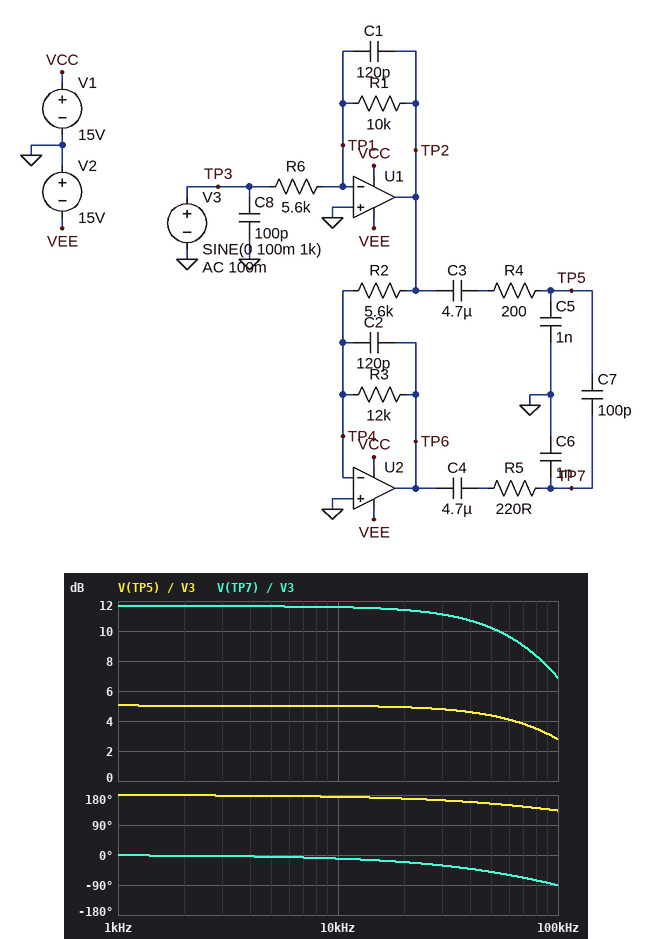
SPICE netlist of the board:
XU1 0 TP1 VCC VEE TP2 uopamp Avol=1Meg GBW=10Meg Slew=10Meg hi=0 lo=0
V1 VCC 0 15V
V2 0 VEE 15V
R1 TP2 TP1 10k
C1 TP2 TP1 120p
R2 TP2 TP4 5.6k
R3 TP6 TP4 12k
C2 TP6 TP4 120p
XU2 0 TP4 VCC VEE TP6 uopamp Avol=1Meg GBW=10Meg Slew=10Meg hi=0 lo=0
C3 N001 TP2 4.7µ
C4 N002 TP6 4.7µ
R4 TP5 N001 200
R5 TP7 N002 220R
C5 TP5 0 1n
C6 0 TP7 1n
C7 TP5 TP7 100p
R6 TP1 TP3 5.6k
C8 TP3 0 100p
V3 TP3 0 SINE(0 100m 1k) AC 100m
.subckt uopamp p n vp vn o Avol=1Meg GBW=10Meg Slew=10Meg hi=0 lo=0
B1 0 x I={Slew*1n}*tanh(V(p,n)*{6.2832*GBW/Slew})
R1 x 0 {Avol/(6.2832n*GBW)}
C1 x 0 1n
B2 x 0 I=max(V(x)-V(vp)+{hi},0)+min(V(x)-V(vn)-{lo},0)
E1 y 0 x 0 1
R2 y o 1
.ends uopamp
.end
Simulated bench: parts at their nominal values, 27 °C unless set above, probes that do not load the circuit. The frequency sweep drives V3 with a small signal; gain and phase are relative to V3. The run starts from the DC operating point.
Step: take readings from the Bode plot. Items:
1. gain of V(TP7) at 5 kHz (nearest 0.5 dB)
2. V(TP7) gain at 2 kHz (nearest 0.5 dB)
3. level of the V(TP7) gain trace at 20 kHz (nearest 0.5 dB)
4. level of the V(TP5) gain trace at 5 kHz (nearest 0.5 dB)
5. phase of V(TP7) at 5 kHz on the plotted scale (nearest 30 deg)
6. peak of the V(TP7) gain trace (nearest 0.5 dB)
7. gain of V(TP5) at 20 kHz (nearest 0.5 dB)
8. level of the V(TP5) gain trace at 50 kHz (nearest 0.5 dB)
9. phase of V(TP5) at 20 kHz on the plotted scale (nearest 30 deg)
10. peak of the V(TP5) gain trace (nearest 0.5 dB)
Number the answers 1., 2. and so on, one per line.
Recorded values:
1. 11.5 dB
2. 11.5 dB
3. 11.5 dB
4. 5.0 dB
5. 0 deg
6. 11.5 dB
7. 5.0 dB
8. 4.5 dB
9. 180 deg
10. 5.0 dB
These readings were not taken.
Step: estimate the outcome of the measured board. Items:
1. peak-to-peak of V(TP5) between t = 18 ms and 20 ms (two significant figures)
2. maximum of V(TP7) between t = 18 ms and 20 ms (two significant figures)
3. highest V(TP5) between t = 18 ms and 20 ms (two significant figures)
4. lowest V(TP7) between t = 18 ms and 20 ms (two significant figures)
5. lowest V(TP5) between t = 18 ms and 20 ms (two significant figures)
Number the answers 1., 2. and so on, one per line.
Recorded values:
1. 360 mV
2. 380 mV
3. 180 mV
4. -380 mV
5. -180 mV
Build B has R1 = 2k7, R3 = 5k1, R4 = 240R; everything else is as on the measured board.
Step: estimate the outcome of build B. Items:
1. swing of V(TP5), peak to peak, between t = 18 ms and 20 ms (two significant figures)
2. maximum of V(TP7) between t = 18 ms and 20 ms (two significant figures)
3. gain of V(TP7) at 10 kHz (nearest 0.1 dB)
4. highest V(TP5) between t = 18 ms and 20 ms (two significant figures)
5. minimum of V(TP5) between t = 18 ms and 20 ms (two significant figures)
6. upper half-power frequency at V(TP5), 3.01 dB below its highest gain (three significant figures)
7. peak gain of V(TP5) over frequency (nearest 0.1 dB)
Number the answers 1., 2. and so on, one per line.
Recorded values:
1. 96 mV
2. 44 mV
3. -7.2 dB
4. 48 mV
5. -48 mV
6. 327 kHz
7. -6.3 dB
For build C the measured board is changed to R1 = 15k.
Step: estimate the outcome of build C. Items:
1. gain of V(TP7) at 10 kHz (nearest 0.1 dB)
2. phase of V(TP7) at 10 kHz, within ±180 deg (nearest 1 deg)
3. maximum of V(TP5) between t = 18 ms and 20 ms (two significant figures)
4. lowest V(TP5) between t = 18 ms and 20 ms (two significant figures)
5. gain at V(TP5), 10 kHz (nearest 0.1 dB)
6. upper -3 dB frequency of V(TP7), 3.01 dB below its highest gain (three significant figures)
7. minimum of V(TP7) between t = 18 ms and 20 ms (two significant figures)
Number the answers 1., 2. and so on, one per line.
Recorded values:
1. 15.1 dB
2. -13 deg
3. 270 mV
4. -270 mV
5. 8.5 dB
6. 61.3 kHz
7. -570 mV
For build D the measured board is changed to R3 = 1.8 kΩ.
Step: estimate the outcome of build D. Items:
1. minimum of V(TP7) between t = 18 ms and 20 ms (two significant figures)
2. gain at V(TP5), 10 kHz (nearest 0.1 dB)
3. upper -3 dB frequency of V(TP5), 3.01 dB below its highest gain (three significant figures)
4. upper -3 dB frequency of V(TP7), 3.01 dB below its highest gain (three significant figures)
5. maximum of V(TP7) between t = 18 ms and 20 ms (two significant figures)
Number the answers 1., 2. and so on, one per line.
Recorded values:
1. -57 mV
2. 5.0 dB
3. 125 kHz
4. 122 kHz
5. 57 mV
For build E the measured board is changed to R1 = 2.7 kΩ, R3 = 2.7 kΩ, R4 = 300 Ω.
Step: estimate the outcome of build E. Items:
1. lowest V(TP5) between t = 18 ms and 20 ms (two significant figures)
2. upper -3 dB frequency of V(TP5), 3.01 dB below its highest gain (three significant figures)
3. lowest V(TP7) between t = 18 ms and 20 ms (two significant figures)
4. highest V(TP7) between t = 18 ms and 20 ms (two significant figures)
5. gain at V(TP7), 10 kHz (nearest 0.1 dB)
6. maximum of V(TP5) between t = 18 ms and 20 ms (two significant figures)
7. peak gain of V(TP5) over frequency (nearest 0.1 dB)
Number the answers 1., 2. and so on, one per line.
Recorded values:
1. -48 mV
2. 299 kHz
3. -23 mV
4. 23 mV
5. -12.7 dB
6. 48 mV
7. -6.3 dB
